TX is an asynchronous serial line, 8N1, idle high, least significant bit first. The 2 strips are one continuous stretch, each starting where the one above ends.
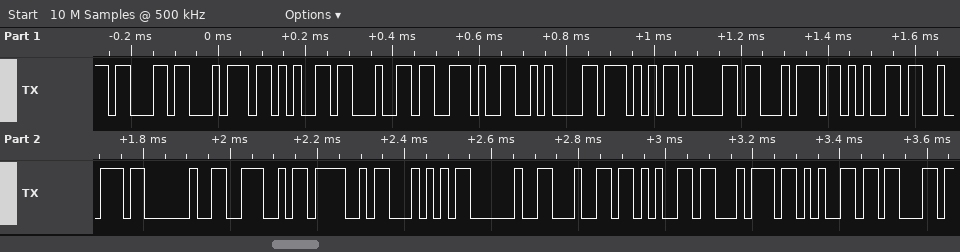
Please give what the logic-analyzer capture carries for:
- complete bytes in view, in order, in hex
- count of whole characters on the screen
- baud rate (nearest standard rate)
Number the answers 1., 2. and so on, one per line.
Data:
1. 63 74 65 64 2E 0A 57 61 74 65 72 20 4E 4F 54 20 64 65 74 65 63
2. 21
3. 57600 baud
